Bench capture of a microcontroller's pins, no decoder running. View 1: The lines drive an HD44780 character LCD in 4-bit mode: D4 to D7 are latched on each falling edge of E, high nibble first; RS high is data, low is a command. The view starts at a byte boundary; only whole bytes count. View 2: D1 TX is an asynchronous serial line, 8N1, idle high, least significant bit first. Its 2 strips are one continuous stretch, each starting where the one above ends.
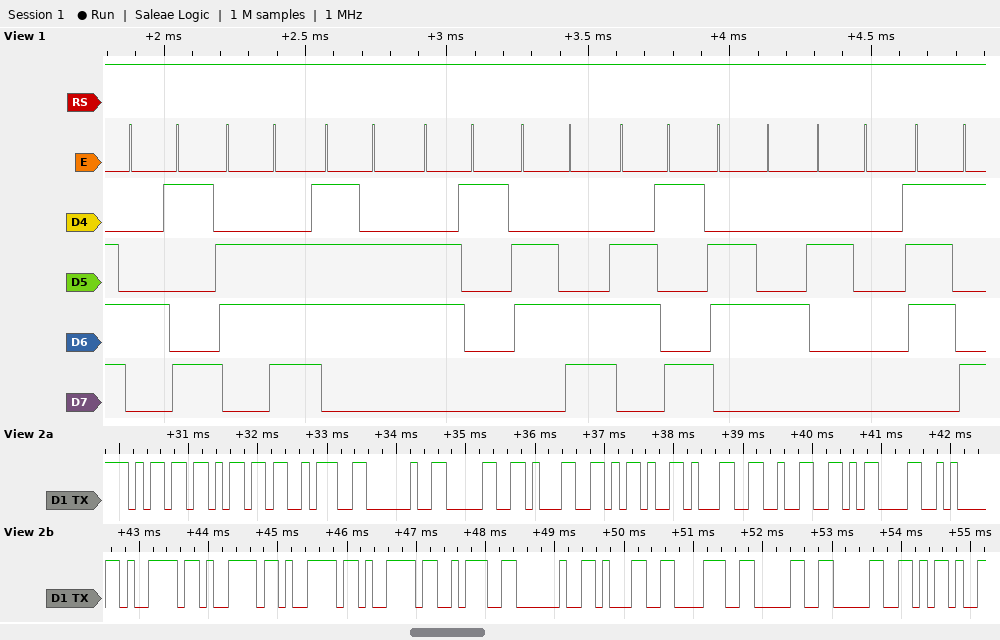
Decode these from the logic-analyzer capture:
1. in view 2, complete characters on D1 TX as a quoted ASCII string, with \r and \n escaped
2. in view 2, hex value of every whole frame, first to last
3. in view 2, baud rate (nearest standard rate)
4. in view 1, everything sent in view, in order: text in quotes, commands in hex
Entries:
"mm: 01-12\r\nyyyy: 1800-"
6D 6D 3A 20 30 31 2D 31 32 0D 0A 79 79 79 79 3A 20 31 38 30 30 2D
9600 baud
"Invalid y"
